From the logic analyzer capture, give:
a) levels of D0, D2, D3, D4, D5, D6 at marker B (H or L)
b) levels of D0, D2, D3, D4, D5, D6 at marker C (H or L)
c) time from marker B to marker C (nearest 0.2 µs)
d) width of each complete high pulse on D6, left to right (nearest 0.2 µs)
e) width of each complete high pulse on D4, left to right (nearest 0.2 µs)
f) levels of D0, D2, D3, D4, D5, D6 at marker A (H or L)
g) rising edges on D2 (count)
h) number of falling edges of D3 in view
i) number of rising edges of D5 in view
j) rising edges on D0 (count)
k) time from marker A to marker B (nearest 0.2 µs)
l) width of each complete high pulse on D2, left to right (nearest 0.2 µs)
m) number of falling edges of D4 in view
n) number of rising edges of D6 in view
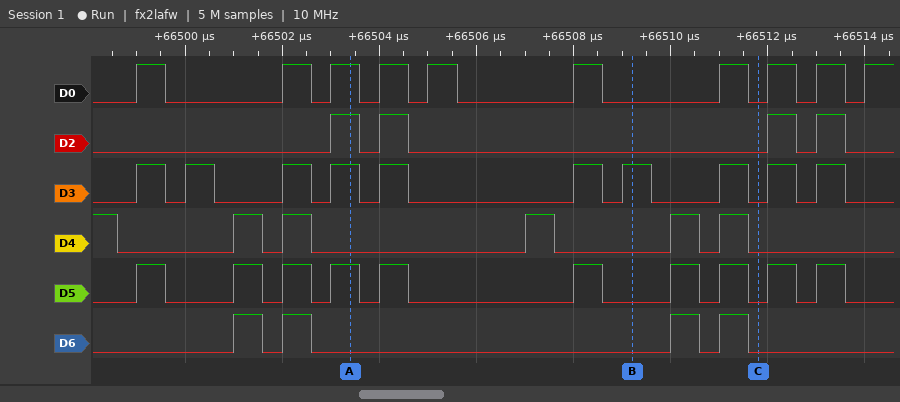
D0=L, D2=L, D3=H, D4=L, D5=L, D6=L
D0=L, D2=L, D3=L, D4=L, D5=L, D6=L
2.6 µs
0.6 µs, 0.6 µs, 0.6 µs, 0.6 µs
0.6 µs, 0.6 µs, 0.6 µs, 0.6 µs, 0.6 µs
D0=H, D2=H, D3=H, D4=L, D5=H, D6=L
4
10
10
10
5.8 µs
0.6 µs, 0.6 µs, 0.6 µs, 0.6 µs
6
4
